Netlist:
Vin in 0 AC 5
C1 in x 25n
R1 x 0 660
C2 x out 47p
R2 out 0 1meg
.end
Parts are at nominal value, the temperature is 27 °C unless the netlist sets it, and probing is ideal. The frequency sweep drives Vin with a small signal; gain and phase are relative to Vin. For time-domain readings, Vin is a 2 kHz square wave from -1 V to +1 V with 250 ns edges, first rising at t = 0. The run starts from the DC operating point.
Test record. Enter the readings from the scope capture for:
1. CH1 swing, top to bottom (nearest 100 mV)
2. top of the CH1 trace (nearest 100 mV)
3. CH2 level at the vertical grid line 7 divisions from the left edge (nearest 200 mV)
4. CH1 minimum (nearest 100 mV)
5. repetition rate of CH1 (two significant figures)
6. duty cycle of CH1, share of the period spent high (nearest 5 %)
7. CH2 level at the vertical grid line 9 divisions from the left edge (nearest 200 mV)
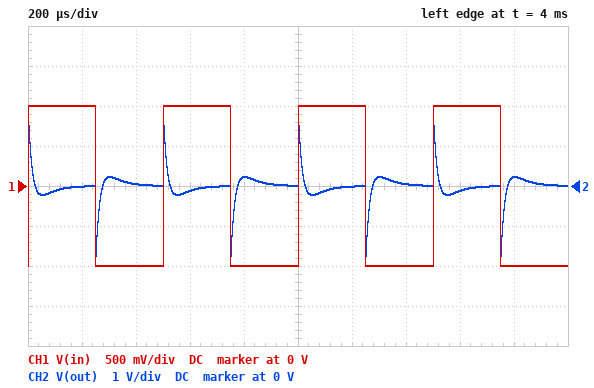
2.0 V
1.0 V
0 V
-1.0 V
2.0 kHz
50 %
200 mV
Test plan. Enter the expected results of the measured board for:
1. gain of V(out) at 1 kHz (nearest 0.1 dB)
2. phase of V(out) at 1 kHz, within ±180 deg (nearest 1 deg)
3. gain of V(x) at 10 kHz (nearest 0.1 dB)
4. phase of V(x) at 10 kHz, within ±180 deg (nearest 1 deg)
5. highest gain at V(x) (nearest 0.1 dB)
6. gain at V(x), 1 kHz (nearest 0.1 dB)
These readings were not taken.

-30.7 dB
158 deg
-2.9 dB
44 deg
0 dB
-19.7 dB
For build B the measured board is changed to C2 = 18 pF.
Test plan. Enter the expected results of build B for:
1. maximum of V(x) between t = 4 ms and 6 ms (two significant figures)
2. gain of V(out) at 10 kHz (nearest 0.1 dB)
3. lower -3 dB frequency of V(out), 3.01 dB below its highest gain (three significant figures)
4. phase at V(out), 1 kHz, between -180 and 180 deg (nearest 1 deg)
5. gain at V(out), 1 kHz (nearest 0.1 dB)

2.0 V
-5.4 dB
14.4 kHz
168 deg
-38.7 dB
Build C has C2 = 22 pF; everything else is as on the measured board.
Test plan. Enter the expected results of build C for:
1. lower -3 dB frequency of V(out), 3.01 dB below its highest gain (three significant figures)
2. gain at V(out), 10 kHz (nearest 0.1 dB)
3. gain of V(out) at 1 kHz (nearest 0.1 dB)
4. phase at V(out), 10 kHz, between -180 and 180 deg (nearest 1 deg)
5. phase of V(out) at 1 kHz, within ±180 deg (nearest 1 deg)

13.2 kHz
-4.7 dB
-37.0 dB
80 deg
166 deg
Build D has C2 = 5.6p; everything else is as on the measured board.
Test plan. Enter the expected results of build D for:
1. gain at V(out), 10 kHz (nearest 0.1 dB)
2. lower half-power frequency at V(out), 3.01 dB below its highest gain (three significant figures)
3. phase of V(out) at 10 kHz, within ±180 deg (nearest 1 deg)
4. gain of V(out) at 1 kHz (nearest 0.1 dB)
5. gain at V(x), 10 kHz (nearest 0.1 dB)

-12.4 dB
31.3 kHz
115 deg
-48.8 dB
-2.9 dB
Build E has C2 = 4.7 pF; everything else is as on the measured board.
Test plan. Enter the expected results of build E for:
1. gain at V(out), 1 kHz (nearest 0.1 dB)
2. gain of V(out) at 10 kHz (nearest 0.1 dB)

-50.3 dB
-13.8 dB
